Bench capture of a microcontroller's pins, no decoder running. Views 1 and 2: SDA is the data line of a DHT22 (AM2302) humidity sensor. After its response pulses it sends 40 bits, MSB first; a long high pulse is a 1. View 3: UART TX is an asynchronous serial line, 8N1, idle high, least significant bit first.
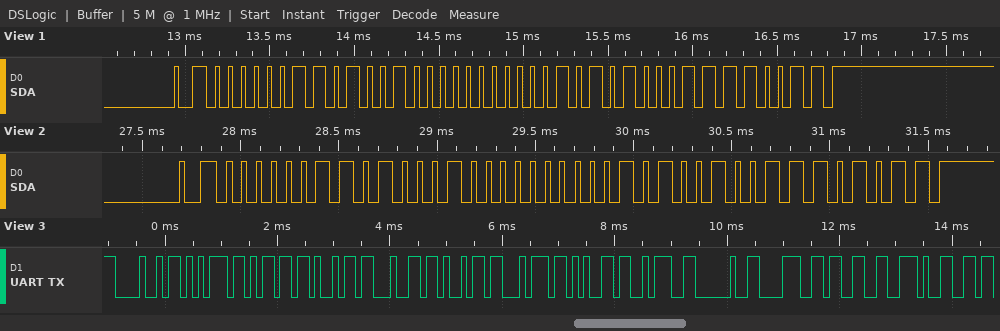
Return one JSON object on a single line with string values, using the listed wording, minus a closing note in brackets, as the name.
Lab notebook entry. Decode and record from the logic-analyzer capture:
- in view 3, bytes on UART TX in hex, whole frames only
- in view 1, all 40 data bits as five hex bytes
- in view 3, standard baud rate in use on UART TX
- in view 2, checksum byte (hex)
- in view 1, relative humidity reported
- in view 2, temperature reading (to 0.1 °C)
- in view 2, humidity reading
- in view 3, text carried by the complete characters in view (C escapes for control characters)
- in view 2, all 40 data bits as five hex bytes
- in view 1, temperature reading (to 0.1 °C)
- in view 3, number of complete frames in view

{"in view 3, bytes on UART TX in hex, whole frames only": "48 75 6D 69 64 69 74 65 3A 20 38 33 2E", "in view 1, all 40 data bits as five hex bytes": "03 48 00 A8 F3", "in view 3, standard baud rate in use on UART TX": "9600 baud", "in view 2, checksum byte": "0xEB", "in view 1, relative humidity reported": "84.0 %", "in view 2, temperature reading": "16.4 °C", "in view 2, humidity reading": "83.6 %", "in view 3, text carried by the complete characters in view": "\"Humidite: 83.\"", "in view 2, all 40 data bits as five hex bytes": "03 44 00 A4 EB", "in view 1, temperature reading": "16.8 °C", "in view 3, number of complete frames in view": "13"}
